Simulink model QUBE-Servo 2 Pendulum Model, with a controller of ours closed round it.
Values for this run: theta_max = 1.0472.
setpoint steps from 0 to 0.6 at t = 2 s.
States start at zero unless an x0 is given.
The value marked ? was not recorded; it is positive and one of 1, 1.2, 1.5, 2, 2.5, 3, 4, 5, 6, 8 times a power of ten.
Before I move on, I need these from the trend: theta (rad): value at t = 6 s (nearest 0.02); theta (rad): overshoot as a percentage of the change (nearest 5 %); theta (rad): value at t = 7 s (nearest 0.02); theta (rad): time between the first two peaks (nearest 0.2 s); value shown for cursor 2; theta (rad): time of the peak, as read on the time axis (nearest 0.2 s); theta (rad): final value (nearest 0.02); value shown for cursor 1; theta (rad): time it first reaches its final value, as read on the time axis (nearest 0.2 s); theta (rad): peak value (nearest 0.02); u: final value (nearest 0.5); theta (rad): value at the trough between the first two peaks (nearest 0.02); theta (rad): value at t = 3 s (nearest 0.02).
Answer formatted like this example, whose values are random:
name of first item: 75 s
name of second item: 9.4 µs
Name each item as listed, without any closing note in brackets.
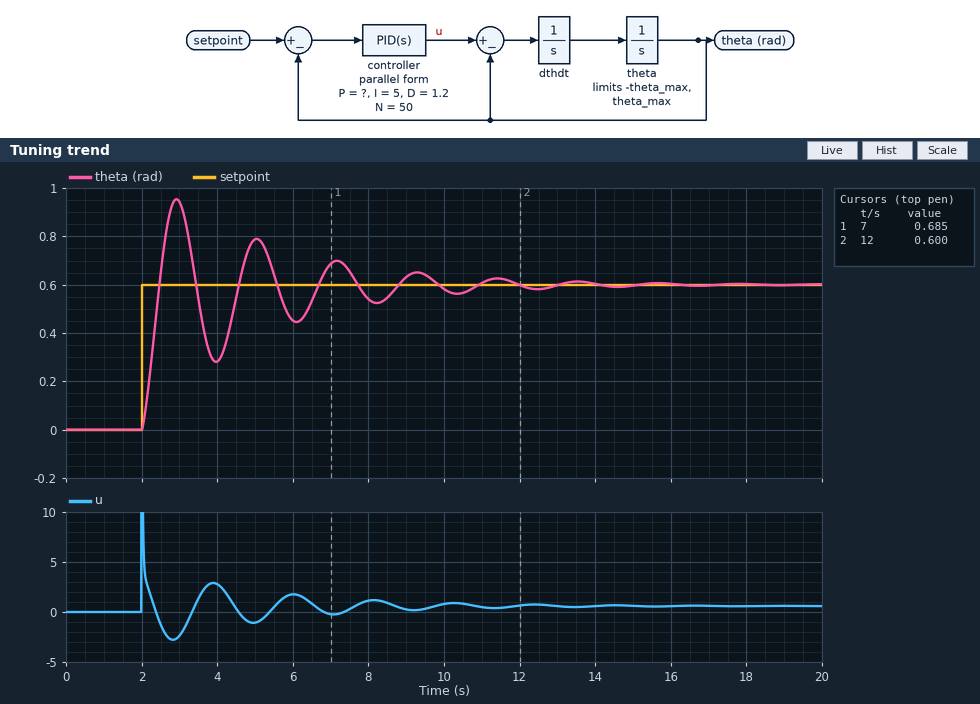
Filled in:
theta (rad): value at t = 6 s: 0.46
theta (rad): overshoot as a percentage of the change: 60 %
theta (rad): value at t = 7 s: 0.68
theta (rad): time between the first two peaks: 2.2 s
value shown for cursor 2: 0.600
theta (rad): time of the peak, as read on the time axis: 3.0 s
theta (rad): final value: 0.60
value shown for cursor 1: 0.685
theta (rad): time it first reaches its final value, as read on the time axis: 2.4 s
theta (rad): peak value: 0.96
u: final value: 0.5
theta (rad): value at the trough between the first two peaks: 0.28
theta (rad): value at t = 3 s: 0.94
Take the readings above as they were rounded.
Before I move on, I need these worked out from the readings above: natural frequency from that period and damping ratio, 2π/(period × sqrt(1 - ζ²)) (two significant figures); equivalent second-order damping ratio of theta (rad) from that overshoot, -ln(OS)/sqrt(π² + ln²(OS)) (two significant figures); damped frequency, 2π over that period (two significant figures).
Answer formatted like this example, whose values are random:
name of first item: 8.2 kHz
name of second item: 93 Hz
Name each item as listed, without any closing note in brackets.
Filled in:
natural frequency from that period and damping ratio, 2π/(period × sqrt(1 - ζ²)): 2.9 rad/s
equivalent second-order damping ratio of theta (rad) from that overshoot, -ln(OS)/sqrt(π² + ln²(OS)): 0.16
damped frequency, 2π over that period: 2.9 rad/s
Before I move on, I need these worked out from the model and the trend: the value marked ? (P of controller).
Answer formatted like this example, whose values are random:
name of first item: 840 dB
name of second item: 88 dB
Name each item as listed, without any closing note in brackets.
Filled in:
the value marked ?: 8
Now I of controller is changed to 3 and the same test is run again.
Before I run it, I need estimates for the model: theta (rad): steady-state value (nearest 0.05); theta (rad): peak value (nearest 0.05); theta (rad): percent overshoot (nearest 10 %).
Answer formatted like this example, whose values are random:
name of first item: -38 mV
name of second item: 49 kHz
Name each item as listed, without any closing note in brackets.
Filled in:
theta (rad): steady-state value: 0.60
theta (rad): peak value: 0.90
theta (rad): percent overshoot: 50 %
